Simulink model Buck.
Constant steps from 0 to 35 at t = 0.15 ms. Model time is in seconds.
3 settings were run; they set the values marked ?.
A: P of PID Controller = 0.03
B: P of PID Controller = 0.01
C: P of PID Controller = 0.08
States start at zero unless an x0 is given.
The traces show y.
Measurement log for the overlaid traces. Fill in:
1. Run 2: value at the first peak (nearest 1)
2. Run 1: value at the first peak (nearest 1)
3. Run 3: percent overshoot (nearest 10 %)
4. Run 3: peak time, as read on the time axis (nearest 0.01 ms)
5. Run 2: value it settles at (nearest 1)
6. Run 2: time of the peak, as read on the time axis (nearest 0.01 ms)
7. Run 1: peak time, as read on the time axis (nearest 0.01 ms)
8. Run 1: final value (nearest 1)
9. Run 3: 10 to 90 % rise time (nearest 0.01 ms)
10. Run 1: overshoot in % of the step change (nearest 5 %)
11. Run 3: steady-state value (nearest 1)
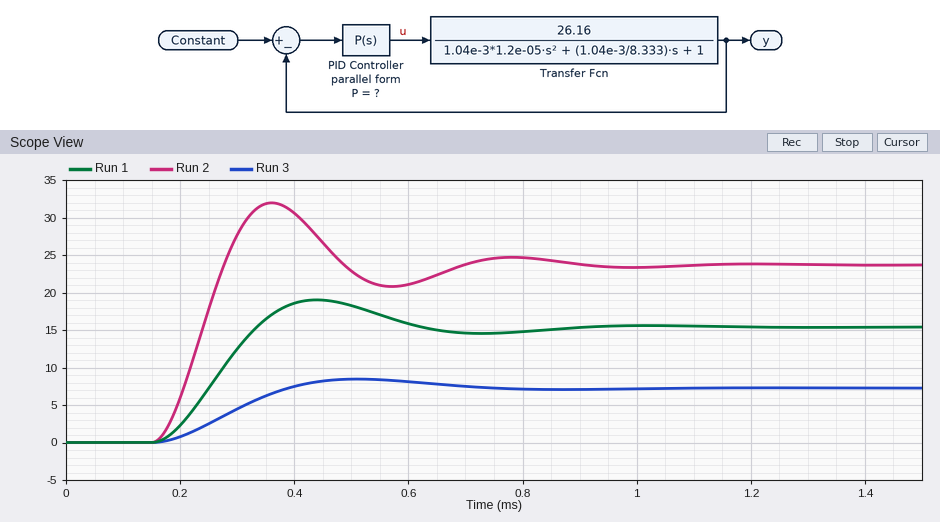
32
19
20 %
0.51 ms
24
0.36 ms
0.44 ms
15
0.16 ms
25 %
7
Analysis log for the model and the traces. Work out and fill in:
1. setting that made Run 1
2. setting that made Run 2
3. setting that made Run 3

A
C
B
